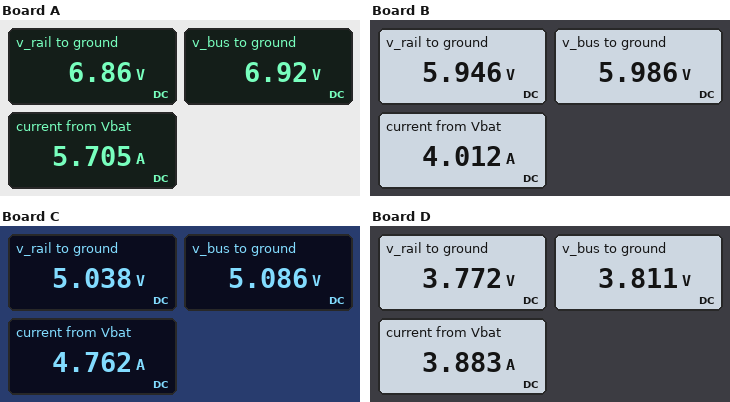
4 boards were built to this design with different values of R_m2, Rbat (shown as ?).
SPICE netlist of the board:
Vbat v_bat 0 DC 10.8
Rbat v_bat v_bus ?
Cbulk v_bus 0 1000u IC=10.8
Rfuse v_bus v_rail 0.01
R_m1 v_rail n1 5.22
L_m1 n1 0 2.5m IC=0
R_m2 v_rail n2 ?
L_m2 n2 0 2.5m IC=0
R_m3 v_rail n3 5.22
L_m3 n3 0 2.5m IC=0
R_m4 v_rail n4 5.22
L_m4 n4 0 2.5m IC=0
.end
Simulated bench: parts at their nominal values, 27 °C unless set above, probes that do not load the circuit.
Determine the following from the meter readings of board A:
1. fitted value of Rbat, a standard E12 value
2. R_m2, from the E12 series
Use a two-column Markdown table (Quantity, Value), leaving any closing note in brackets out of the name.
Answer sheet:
| Quantity | Value |
|---|---|
| fitted value of Rbat, a standard E12 value | 0.68 Ω |
| R_m2, from the E12 series | 3.9 Ω |
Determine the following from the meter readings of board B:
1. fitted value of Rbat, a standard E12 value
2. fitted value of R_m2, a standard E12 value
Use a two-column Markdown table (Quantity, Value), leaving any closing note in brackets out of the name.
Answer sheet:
| Quantity | Value |
|---|---|
| fitted value of Rbat, a standard E12 value | 1.2 Ω |
| fitted value of R_m2, a standard E12 value | 10 Ω |
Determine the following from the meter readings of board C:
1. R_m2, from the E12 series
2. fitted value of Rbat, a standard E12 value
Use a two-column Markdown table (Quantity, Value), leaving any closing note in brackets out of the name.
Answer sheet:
| Quantity | Value |
|---|---|
| R_m2, from the E12 series | 2.7 Ω |
| fitted value of Rbat, a standard E12 value | 1.2 Ω |
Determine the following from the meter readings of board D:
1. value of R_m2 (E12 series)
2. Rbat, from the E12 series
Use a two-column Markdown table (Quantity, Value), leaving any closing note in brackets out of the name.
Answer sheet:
| Quantity | Value |
|---|---|
| value of R_m2 | 2.2 Ω |
| Rbat, from the E12 series | 1.8 Ω |
